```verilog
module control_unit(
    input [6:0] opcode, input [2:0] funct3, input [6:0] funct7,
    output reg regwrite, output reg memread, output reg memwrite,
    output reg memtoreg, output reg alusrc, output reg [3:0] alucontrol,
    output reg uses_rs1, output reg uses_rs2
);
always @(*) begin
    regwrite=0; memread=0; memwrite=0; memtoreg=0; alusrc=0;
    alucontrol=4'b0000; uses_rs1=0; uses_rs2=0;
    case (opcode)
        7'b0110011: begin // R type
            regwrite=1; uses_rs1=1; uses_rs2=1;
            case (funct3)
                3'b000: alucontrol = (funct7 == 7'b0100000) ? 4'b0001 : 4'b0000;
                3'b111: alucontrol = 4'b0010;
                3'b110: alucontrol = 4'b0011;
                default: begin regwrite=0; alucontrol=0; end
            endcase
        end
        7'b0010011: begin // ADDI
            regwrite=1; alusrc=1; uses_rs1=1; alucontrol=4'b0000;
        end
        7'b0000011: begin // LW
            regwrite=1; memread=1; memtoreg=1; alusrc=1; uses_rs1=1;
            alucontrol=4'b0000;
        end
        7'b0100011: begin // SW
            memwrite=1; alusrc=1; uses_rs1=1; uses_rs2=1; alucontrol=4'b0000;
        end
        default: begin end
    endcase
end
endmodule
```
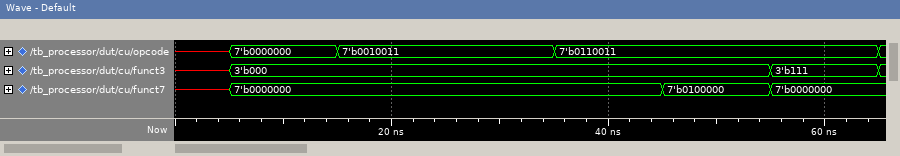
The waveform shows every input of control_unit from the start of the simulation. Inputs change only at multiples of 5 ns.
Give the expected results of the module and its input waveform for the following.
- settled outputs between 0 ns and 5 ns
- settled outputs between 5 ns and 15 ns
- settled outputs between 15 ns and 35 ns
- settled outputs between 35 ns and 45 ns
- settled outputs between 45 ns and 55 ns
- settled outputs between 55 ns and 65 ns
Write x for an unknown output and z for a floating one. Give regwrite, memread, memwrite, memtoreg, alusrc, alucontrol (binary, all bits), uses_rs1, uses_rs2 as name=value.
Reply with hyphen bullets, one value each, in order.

- regwrite=x, memread=x, memwrite=x, memtoreg=x, alusrc=x, alucontrol=x, uses_rs1=x, uses_rs2=x
- regwrite=0, memread=0, memwrite=0, memtoreg=0, alusrc=0, alucontrol=0000, uses_rs1=0, uses_rs2=0
- regwrite=1, memread=0, memwrite=0, memtoreg=0, alusrc=1, alucontrol=0000, uses_rs1=1, uses_rs2=0
- regwrite=1, memread=0, memwrite=0, memtoreg=0, alusrc=0, alucontrol=0000, uses_rs1=1, uses_rs2=1
- regwrite=1, memread=0, memwrite=0, memtoreg=0, alusrc=0, alucontrol=0001, uses_rs1=1, uses_rs2=1
- regwrite=1, memread=0, memwrite=0, memtoreg=0, alusrc=0, alucontrol=0010, uses_rs1=1, uses_rs2=1
